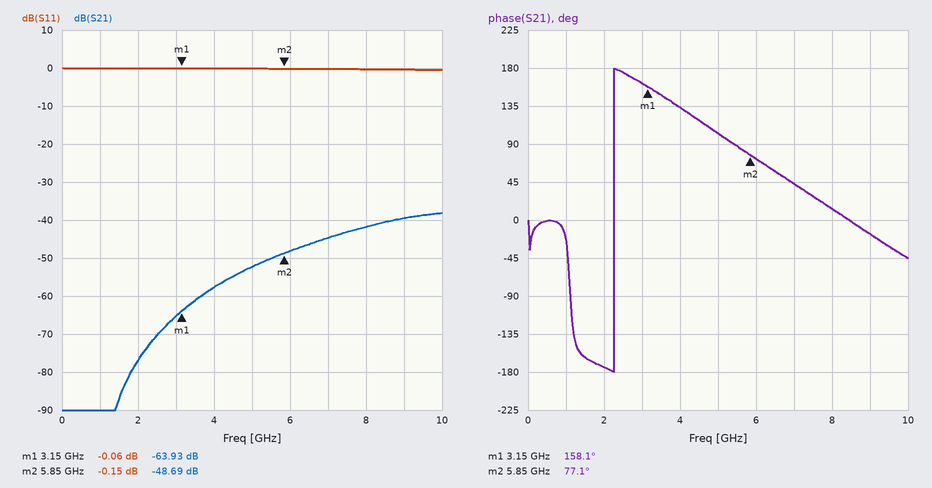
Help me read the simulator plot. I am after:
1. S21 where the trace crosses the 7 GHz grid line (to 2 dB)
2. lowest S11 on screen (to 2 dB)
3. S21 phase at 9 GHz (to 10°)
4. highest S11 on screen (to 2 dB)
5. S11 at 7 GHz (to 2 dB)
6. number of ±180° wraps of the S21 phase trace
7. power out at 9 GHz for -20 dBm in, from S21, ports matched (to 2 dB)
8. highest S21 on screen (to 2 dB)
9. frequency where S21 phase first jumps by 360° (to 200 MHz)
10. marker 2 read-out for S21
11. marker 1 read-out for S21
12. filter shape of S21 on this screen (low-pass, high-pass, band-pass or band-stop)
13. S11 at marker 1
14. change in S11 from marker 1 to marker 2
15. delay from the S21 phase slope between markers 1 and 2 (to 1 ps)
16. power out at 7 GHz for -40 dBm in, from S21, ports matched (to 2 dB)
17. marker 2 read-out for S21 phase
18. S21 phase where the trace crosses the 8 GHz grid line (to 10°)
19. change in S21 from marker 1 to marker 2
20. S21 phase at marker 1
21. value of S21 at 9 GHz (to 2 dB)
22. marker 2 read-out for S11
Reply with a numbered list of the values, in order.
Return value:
1. -44 dB
2. 0 dB
3. -20°
4. 0 dB
5. 0 dB
6. 1
7. -60 dBm
8. -38 dB
9. 2.2 GHz
10. -48.69 dB
11. -63.93 dB
12. high-pass
13. -0.06 dB
14. -0.09 dB
15. 83 ps
16. -84 dBm
17. 77.1°
18. 10°
19. 15.24 dB
20. 158.1°
21. -40 dB
22. -0.15 dB
